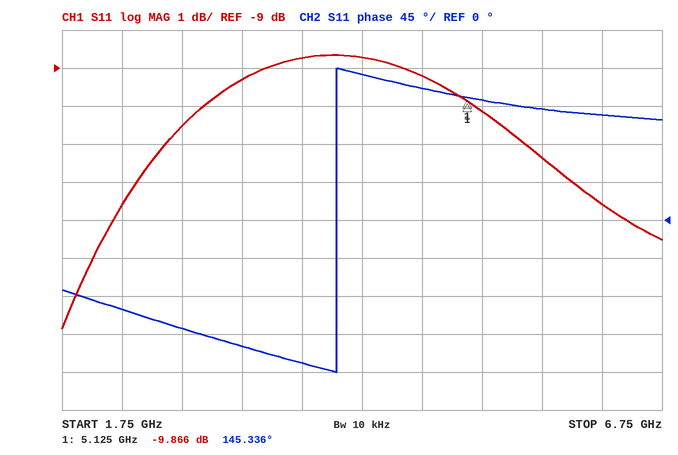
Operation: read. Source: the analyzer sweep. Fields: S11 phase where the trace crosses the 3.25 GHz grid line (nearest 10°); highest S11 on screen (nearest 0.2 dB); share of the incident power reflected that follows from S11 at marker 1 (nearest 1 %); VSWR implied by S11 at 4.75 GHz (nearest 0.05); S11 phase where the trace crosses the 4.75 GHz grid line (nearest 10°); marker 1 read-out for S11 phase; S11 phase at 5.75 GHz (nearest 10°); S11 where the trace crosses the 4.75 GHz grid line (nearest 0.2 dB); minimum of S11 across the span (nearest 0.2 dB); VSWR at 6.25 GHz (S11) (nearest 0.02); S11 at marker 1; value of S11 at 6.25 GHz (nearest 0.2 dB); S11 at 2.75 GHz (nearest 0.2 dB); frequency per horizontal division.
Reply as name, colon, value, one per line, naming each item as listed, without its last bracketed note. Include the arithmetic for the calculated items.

S11 phase where the trace crosses the 3.25 GHz grid line: -150°
highest S11 on screen: -8.6 dB
share of the incident power reflected that follows from S11 at marker 1: 10^(-9.866/10) ≈ 10 %
VSWR implied by S11 at 4.75 GHz: |Γ| = 10^(-9.2/20) = 0.3467; VSWR = (1 + 0.3467)/(1 − 0.3467) ≈ 2.06, so 2.05 to the nearest 0.05
S11 phase where the trace crosses the 4.75 GHz grid line: 160°
marker 1 read-out for S11 phase: 145.336°
S11 phase at 5.75 GHz: 130°
S11 where the trace crosses the 4.75 GHz grid line: -9.2 dB
minimum of S11 across the span: -15.8 dB
VSWR at 6.25 GHz (S11): |Γ| = 10^(-12.6/20) = 0.2344; VSWR = (1 + 0.2344)/(1 − 0.2344) ≈ 1.61, so 1.62 to the nearest 0.02
S11 at marker 1: -9.866 dB
value of S11 at 6.25 GHz: -12.6 dB
S11 at 2.75 GHz: -10.6 dB
frequency per horizontal division: 500 MHz
